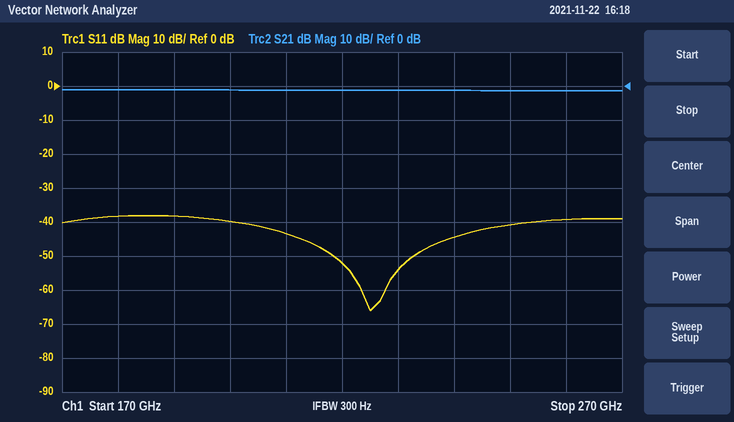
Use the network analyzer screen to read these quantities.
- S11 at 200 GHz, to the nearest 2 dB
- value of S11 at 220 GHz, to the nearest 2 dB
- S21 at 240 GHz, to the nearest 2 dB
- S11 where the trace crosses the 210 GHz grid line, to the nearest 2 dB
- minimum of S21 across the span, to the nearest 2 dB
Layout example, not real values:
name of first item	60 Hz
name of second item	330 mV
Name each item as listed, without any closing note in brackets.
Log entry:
S11 at 200 GHz, to the nearest 2 dB	-40 dB
value of S11 at 220 GHz, to the nearest 2 dB	-52 dB
S21 at 240 GHz, to the nearest 2 dB	-2 dB
S11 where the trace crosses the 210 GHz grid line, to the nearest 2 dB	-44 dB
minimum of S21 across the span, to the nearest 2 dB	-2 dB
